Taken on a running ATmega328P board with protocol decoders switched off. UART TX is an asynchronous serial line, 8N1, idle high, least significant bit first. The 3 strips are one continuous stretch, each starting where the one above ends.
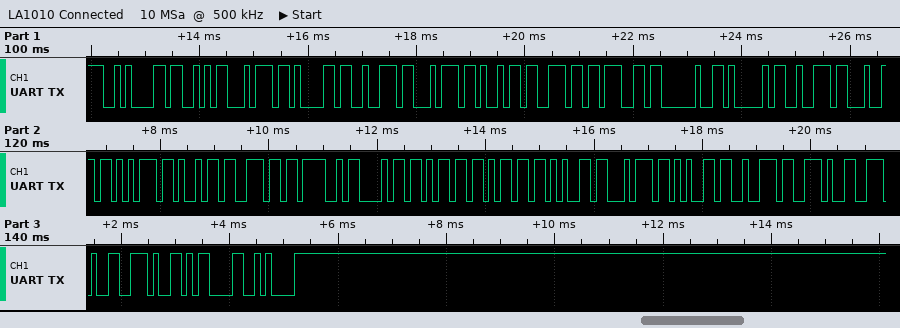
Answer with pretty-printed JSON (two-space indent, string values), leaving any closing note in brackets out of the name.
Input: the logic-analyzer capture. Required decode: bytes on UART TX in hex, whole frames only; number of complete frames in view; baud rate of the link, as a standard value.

{
  "bytes on UART TX in hex, whole frames only": "0x0A 0x53 0x74 0x61 0x72 0x74 0x69 0x6E 0x67 0x20 0x41 0x72 0x64 0x75 0x69 0x6E 0x4F 0x68 0x6D 0x6D 0x65 0x74 0x65 0x72 0x2E 0x2E 0x2E 0x0D 0x0A",
  "number of complete frames in view": "29",
  "baud rate of the link, as a standard value": "9600 baud"
}
